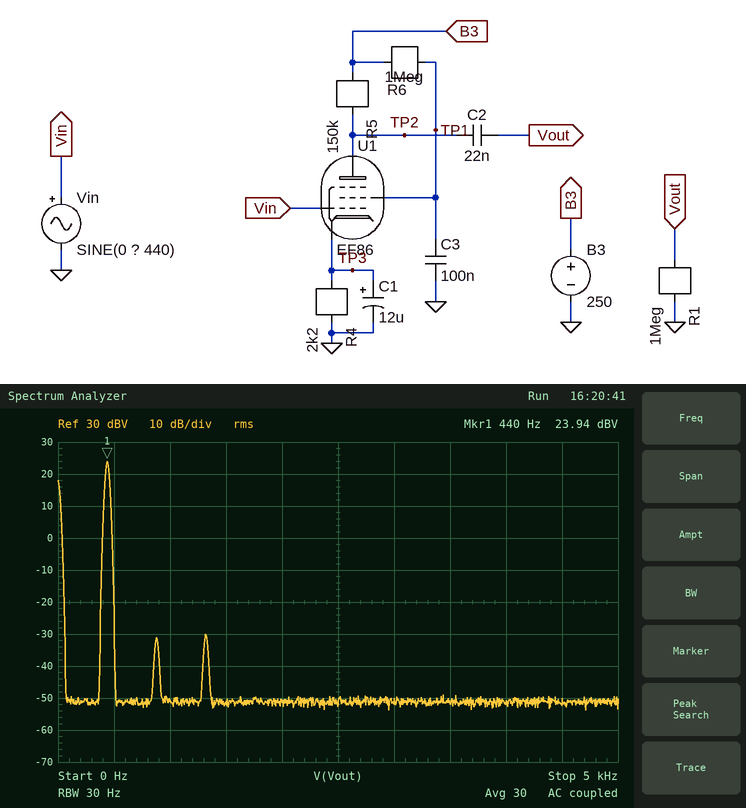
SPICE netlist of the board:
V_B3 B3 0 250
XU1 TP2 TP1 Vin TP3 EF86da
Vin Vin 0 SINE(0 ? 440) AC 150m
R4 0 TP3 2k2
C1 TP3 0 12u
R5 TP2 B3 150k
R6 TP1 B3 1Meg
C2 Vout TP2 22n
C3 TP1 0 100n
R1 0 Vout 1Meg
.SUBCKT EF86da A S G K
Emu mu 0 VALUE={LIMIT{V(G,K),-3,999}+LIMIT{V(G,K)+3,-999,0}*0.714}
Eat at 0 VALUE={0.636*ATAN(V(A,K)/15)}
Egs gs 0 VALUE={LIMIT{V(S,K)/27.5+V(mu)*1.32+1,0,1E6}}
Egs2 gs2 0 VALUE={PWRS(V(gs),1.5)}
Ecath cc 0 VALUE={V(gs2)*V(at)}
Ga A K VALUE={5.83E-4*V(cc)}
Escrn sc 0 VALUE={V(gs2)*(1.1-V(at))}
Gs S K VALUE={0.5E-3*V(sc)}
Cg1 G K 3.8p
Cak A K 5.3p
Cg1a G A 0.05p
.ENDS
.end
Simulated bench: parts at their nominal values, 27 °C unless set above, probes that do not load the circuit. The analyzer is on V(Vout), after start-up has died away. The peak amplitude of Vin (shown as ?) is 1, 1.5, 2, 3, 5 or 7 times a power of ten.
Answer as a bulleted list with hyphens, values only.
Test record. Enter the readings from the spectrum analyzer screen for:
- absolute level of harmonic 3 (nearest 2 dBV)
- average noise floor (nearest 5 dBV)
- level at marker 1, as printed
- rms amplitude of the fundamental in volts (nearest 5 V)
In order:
- -30 dBV
- -50 dBV
- 23.94 dBV
- 15 V
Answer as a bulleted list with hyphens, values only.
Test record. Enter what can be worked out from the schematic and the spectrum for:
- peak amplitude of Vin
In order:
- 150 mV
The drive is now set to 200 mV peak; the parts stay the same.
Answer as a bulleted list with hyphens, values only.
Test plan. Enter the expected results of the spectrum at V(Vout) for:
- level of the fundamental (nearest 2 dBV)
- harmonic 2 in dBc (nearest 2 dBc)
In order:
- 26 dBV
- -52 dBc
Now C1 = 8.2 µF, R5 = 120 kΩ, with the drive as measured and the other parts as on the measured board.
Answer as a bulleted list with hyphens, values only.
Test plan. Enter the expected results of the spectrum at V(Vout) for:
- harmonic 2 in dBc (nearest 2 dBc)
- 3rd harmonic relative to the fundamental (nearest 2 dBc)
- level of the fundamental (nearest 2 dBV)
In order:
- -42 dBc
- -60 dBc
- 22 dBV
